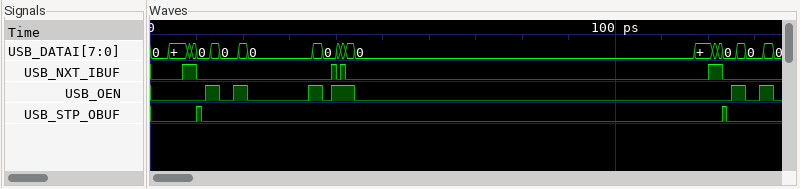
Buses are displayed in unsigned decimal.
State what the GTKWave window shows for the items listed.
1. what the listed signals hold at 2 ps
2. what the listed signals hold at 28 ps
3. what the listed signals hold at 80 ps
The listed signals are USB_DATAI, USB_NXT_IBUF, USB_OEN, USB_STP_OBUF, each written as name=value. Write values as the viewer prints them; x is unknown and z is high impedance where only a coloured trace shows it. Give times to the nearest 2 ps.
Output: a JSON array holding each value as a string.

["USB_DATAI=0, USB_NXT_IBUF=0, USB_OEN=0, USB_STP_OBUF=0", "USB_DATAI=0, USB_NXT_IBUF=0, USB_OEN=0, USB_STP_OBUF=0", "USB_DATAI=0, USB_NXT_IBUF=0, USB_OEN=0, USB_STP_OBUF=0"]
